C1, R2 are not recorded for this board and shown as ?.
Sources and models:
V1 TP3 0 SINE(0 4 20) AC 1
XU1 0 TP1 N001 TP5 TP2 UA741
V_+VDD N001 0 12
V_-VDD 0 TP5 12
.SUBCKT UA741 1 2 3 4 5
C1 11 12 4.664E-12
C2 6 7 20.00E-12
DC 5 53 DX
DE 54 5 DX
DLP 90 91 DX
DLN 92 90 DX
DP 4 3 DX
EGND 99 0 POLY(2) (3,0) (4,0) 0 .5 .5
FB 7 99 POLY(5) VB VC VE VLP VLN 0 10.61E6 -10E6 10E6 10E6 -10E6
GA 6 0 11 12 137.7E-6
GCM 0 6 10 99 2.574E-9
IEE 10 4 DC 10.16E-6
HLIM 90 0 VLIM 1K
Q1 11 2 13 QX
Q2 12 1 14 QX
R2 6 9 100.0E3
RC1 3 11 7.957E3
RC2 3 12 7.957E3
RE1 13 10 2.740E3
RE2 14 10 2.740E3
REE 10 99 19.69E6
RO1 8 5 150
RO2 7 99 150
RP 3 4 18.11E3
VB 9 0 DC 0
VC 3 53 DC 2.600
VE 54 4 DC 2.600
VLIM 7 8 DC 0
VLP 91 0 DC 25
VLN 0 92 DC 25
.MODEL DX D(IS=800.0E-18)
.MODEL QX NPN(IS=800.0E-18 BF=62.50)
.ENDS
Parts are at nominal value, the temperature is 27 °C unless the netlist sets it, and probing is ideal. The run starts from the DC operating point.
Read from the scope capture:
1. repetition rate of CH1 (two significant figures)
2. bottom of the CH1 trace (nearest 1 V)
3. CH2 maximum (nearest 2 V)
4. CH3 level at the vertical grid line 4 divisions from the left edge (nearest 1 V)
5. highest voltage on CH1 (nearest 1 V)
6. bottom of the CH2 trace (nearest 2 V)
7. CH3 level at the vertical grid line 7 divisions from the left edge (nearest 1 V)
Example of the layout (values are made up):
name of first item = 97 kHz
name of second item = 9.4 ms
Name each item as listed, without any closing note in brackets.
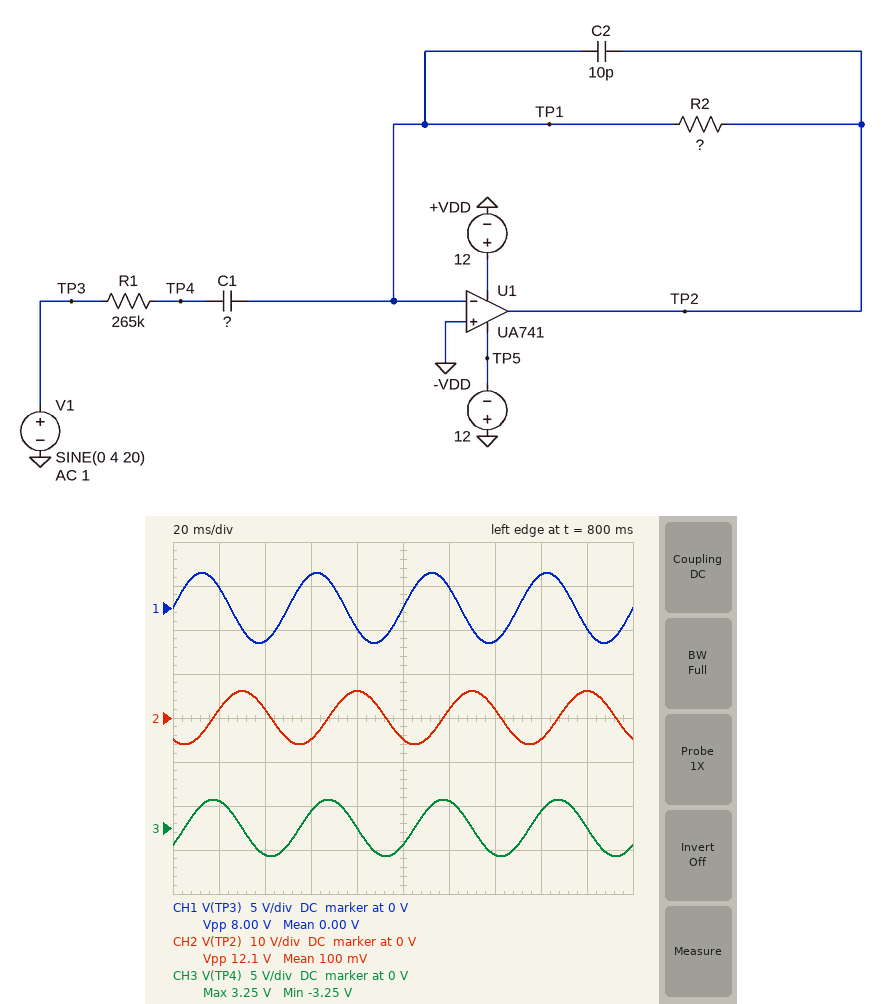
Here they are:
repetition rate of CH1 = 20 Hz
bottom of the CH1 trace = -4 V
CH2 maximum = 6 V
CH3 level at the vertical grid line 4 divisions from the left edge = 0 V
highest voltage on CH1 = 4 V
bottom of the CH2 trace = -6 V
CH3 level at the vertical grid line 7 divisions from the left edge = -3 V
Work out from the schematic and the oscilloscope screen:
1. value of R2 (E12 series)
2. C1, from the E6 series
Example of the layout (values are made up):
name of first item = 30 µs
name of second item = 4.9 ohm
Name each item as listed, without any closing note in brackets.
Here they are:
value of R2 = 680 kΩ
C1, from the E6 series = 22 nF
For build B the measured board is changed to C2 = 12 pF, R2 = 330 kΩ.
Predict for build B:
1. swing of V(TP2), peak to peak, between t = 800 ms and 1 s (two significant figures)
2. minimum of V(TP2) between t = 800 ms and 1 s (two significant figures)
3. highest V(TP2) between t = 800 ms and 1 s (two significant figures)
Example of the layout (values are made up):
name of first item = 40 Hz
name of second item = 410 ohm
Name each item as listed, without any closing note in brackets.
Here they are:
swing of V(TP2), peak to peak, between t = 800 ms and 1 s = 5.9 V
minimum of V(TP2) between t = 800 ms and 1 s = -2.9 V
highest V(TP2) between t = 800 ms and 1 s = 3.0 V
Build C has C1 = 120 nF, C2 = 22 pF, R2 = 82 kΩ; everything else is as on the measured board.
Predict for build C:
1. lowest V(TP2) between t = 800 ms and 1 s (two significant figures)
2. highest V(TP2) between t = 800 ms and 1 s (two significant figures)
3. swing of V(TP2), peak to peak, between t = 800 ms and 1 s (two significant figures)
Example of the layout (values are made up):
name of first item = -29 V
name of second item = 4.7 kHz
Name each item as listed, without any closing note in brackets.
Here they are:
lowest V(TP2) between t = 800 ms and 1 s = -1.2 V
highest V(TP2) between t = 800 ms and 1 s = 1.2 V
swing of V(TP2), peak to peak, between t = 800 ms and 1 s = 2.4 V
